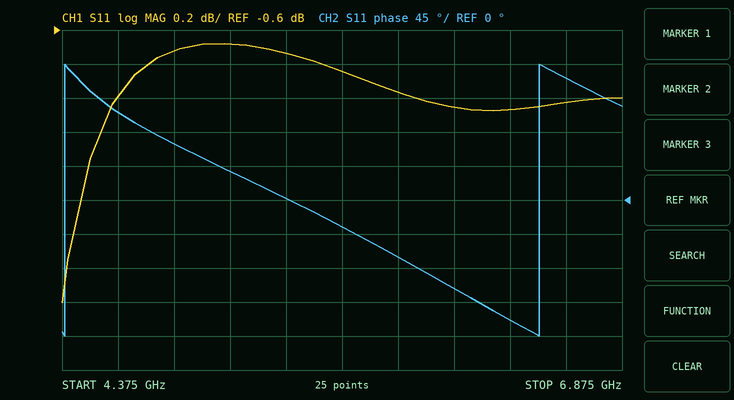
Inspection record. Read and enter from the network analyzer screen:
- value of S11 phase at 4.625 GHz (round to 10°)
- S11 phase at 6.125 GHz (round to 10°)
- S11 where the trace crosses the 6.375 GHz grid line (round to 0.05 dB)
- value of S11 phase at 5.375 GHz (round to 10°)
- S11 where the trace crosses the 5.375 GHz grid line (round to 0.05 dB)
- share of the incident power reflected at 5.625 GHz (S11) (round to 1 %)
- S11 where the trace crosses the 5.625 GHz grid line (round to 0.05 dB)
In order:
120°
-120°
-1.05 dB
0°
-0.75 dB
82 %
-0.85 dB
